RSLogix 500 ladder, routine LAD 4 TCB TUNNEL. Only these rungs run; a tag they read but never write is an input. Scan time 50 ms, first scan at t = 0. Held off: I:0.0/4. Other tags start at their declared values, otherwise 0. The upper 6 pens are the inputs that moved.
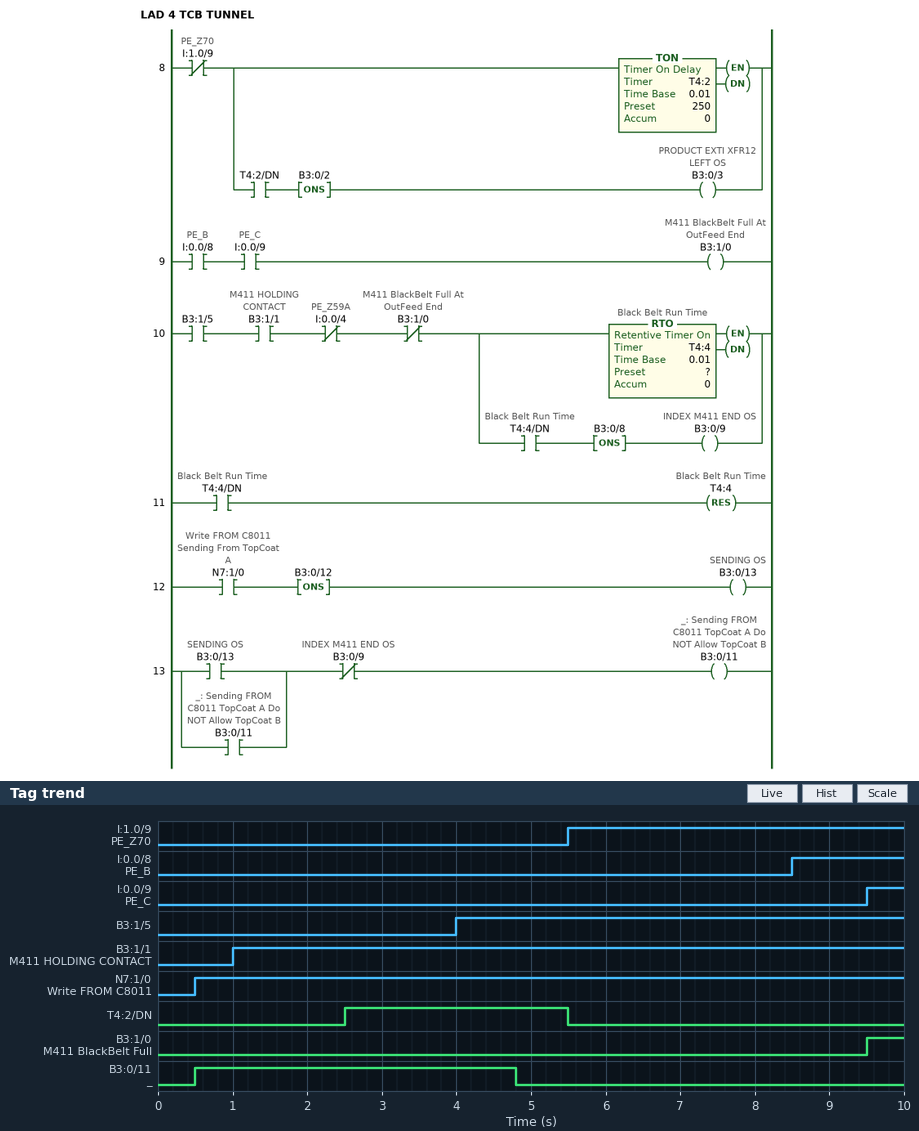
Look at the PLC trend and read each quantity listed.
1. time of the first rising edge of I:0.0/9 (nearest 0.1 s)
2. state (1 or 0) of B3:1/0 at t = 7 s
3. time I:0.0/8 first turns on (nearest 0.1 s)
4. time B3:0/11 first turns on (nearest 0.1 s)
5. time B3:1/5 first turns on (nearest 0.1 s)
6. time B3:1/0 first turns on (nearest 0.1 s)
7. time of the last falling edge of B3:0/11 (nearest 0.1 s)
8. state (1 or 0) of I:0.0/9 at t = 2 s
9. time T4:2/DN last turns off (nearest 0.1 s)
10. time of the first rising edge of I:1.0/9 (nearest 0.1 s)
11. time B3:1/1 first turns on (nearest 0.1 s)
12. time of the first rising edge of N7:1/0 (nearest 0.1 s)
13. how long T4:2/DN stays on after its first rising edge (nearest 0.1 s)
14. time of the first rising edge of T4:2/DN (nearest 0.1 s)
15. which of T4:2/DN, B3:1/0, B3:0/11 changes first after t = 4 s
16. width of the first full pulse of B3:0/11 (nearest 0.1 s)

9.5 s
0
8.5 s
0.5 s
4.0 s
9.5 s
4.8 s
0
5.5 s
5.5 s
1.0 s
0.5 s
3.0 s
2.5 s
B3:0/11
4.3 s
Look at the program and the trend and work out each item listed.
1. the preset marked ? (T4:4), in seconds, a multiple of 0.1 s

0.8 s
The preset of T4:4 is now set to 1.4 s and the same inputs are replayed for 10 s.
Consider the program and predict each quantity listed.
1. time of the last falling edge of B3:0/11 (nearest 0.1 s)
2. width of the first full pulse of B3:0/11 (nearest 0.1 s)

5.4 s
4.9 s
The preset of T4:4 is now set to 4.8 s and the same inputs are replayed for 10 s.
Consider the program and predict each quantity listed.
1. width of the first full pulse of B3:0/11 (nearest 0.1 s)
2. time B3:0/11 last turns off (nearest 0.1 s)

8.3 s
8.8 s
